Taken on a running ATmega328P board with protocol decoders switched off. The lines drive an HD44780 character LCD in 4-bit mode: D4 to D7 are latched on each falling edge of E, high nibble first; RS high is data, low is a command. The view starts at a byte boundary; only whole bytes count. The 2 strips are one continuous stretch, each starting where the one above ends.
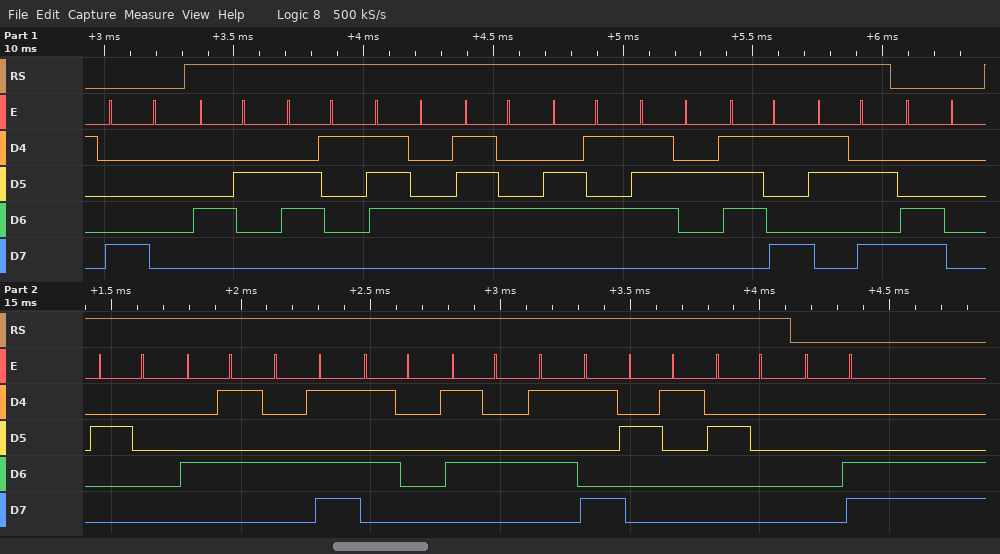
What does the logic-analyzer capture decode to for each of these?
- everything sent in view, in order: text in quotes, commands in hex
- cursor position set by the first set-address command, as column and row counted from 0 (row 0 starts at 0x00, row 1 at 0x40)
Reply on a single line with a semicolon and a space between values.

0x80 "Battery:" 0xC0 " EMPTY! " 0x0C; column 0, row 0
